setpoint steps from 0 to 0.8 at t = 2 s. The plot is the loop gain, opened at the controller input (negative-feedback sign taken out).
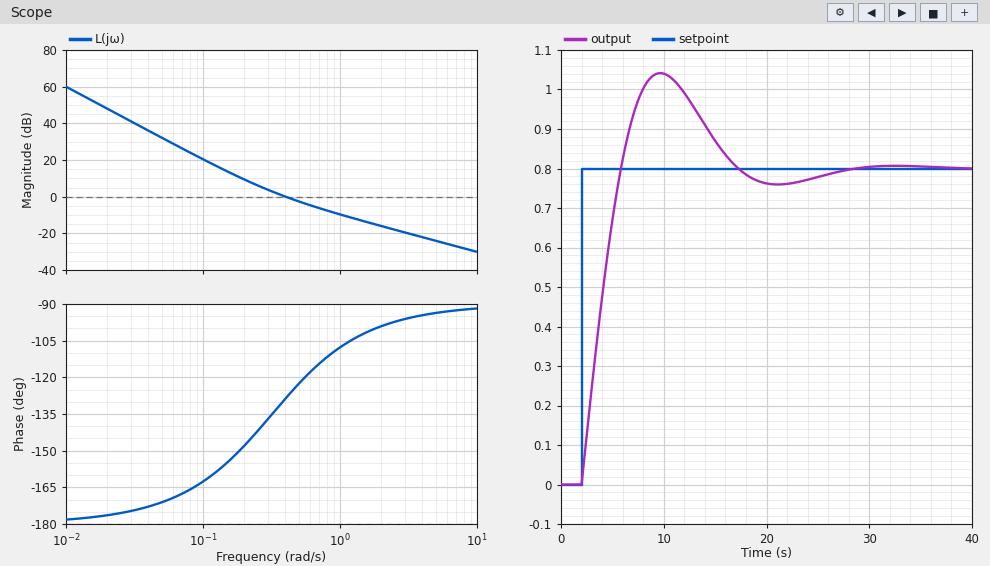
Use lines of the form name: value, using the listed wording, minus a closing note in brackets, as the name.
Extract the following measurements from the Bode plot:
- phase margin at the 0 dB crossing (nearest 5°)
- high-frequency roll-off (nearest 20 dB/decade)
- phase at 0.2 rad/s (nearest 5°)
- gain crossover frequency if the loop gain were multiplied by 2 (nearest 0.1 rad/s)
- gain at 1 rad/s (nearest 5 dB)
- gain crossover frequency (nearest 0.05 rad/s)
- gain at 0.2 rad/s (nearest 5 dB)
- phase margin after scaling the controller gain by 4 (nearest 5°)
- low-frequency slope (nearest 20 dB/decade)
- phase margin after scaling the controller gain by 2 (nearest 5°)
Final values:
phase margin at the 0 dB crossing: 50°
high-frequency roll-off: -20 dB/decade
phase at 0.2 rad/s: -150°
gain crossover frequency if the loop gain were multiplied by 2: 0.7 rad/s
gain at 1 rad/s: -10 dB
gain crossover frequency: 0.40 rad/s
gain at 0.2 rad/s: 10 dB
phase margin after scaling the controller gain by 4: 75°
low-frequency slope: -40 dB/decade
phase margin after scaling the controller gain by 2: 65°
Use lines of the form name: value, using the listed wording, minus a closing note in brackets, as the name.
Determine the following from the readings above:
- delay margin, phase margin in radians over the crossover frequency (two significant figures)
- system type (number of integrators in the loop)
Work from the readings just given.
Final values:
delay margin, phase margin in radians over the crossover frequency: 2.2 s
system type: 2
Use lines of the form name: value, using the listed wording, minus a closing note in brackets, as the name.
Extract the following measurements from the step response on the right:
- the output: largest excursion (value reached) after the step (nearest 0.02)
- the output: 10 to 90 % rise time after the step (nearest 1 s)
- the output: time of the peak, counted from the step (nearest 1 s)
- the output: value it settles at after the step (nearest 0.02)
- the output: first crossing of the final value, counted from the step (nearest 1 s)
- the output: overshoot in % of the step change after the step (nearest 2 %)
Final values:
the output: largest excursion (value reached) after the step: 1.04
the output: 10 to 90 % rise time after the step: 3 s
the output: time of the peak, counted from the step: 8 s
the output: value it settles at after the step: 0.80
the output: first crossing of the final value, counted from the step: 4 s
the output: overshoot in % of the step change after the step: 30 %
